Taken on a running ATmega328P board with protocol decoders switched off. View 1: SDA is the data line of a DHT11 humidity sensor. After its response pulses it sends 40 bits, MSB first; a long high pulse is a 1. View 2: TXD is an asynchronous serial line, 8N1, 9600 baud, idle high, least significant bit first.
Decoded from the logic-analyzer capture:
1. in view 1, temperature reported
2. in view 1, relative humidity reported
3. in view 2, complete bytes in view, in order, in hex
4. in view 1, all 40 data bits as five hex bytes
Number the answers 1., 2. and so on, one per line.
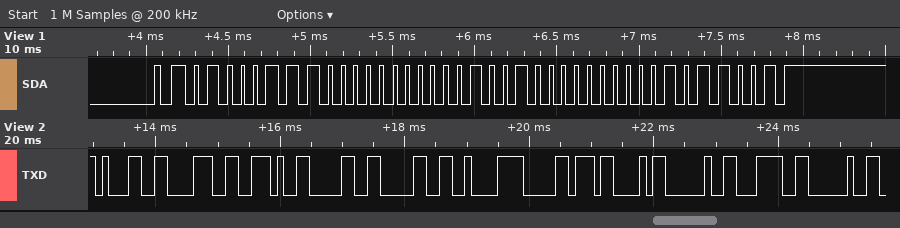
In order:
1. 18.0 °C
2. 71 %
3. 0x31 0x38 0x2E 0x30 0x30 0xC2 0xB0 0x43 0x20 0x3C 0x20
4. 47 00 12 00 59
